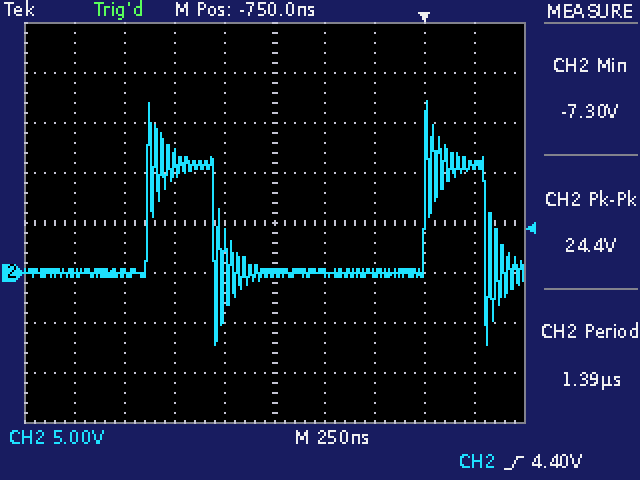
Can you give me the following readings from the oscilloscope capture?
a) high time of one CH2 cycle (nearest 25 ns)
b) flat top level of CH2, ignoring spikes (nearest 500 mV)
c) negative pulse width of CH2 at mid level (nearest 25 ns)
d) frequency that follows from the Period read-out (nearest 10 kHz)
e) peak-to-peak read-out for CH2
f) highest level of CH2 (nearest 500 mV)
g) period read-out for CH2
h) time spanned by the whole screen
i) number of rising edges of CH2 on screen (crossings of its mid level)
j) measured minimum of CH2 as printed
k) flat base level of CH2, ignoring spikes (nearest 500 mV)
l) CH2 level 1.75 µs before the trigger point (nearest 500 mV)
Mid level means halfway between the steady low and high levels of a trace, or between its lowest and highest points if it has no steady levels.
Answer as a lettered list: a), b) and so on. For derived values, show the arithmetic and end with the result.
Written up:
a) 325 ns
b) 11.0 V
c) 1.075 µs
d) 1 / 1.39 µs ≈ 719 kHz, so 720 kHz to the nearest 10 kHz
e) 24.4 V
f) 17.0 V
g) 1.39 µs
h) 2.5 µs
i) 2
j) -7.30 V
k) 0.0 V
l) 0.0 V
